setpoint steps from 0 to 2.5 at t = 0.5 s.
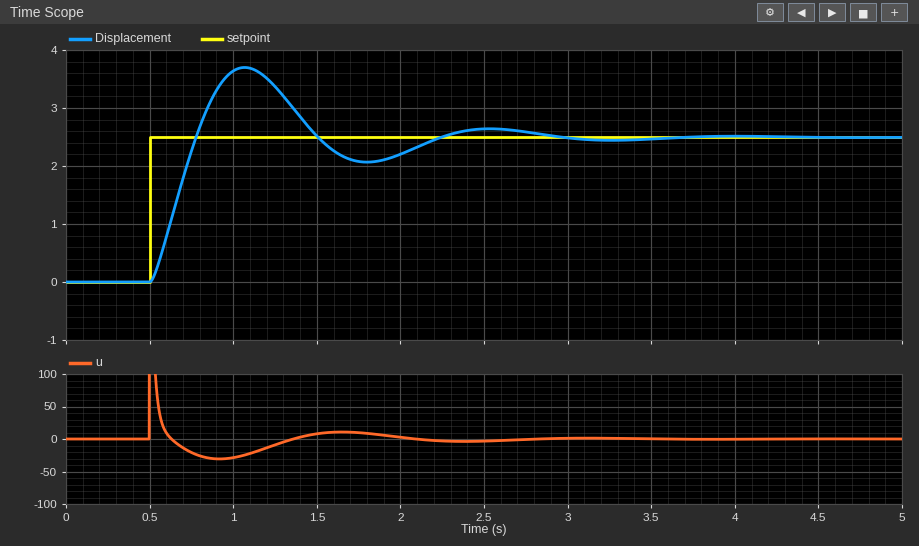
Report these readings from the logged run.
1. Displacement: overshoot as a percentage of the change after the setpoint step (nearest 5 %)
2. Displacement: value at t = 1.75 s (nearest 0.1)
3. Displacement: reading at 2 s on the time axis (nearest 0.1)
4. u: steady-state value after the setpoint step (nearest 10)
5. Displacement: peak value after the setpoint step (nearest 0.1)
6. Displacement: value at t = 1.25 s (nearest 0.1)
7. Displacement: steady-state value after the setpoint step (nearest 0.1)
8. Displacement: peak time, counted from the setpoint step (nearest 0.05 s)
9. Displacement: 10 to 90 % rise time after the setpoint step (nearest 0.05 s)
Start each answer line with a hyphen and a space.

- 50 %
- 2.1
- 2.2
- 0
- 3.7
- 3.4
- 2.5
- 0.55 s
- 0.20 s
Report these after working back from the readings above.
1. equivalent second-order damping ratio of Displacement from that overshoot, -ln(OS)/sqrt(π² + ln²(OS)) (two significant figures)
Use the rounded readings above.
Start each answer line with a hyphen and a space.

- 0.22
